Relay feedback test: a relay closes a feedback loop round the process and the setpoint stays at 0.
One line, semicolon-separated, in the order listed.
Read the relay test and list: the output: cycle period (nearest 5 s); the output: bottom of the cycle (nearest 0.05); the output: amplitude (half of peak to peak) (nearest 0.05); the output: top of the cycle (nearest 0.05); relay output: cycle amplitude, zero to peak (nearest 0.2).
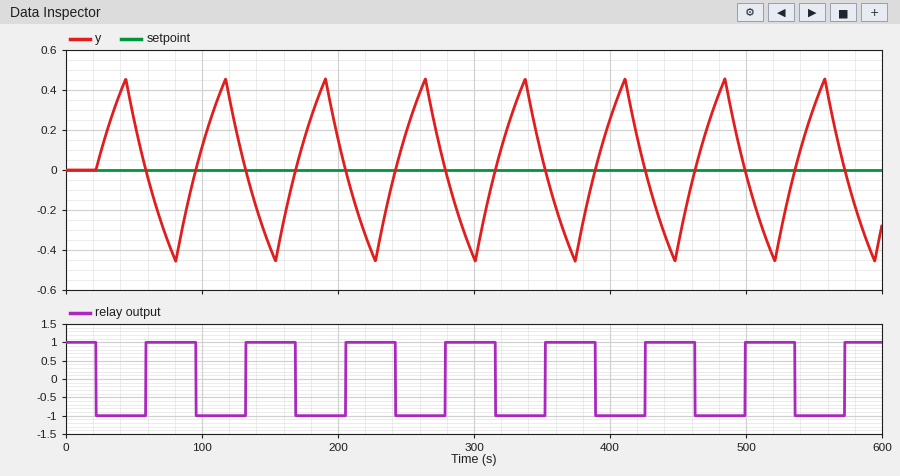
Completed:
75 s; -0.45; 0.45; 0.45; 1.0
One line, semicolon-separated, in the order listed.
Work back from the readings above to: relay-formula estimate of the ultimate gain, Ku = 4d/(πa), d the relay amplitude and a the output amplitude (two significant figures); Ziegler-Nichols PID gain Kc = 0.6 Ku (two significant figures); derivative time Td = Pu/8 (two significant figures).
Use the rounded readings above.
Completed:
2.8; 1.7; 9.4 s
